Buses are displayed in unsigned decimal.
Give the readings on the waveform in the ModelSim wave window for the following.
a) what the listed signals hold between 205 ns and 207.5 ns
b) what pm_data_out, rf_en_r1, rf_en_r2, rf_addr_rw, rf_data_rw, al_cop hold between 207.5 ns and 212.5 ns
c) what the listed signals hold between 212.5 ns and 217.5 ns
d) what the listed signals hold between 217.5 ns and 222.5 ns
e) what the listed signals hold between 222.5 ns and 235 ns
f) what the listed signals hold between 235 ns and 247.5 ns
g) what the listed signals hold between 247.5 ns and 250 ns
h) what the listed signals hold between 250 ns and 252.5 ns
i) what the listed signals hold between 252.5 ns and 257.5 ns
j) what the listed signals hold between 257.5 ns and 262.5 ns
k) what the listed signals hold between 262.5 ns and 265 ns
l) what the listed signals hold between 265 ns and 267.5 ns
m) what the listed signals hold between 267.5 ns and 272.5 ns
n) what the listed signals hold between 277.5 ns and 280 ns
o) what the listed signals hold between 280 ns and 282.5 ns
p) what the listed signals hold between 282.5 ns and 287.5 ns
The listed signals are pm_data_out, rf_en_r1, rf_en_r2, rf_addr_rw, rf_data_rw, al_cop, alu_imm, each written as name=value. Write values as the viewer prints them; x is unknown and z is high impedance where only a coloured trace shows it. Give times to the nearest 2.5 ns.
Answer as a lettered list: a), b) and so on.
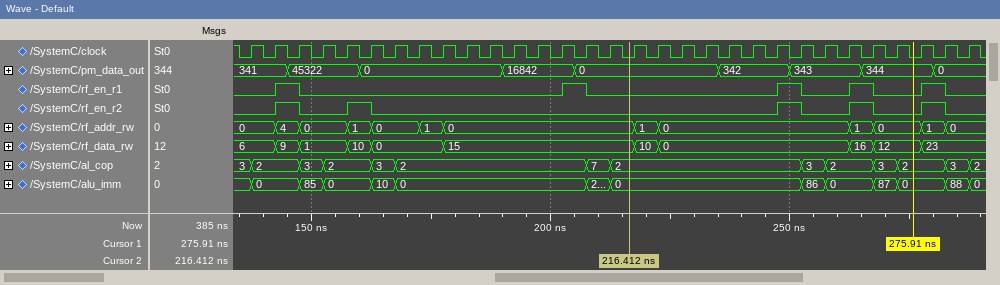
a) pm_data_out=0, rf_en_r1=1, rf_en_r2=0, rf_addr_rw=0, rf_data_rw=15, al_cop=2, alu_imm=0
b) pm_data_out=0, rf_en_r1=0, rf_en_r2=0, rf_addr_rw=0, rf_data_rw=15, al_cop=7
c) pm_data_out=0, rf_en_r1=0, rf_en_r2=0, rf_addr_rw=0, rf_data_rw=15, al_cop=2, alu_imm=0
d) pm_data_out=0, rf_en_r1=0, rf_en_r2=0, rf_addr_rw=1, rf_data_rw=10, al_cop=2, alu_imm=0
e) pm_data_out=0, rf_en_r1=0, rf_en_r2=0, rf_addr_rw=0, rf_data_rw=0, al_cop=2, alu_imm=0
f) pm_data_out=342, rf_en_r1=0, rf_en_r2=0, rf_addr_rw=0, rf_data_rw=0, al_cop=2, alu_imm=0
g) pm_data_out=342, rf_en_r1=1, rf_en_r2=1, rf_addr_rw=0, rf_data_rw=0, al_cop=2, alu_imm=0
h) pm_data_out=343, rf_en_r1=1, rf_en_r2=1, rf_addr_rw=0, rf_data_rw=0, al_cop=2, alu_imm=0
i) pm_data_out=343, rf_en_r1=0, rf_en_r2=0, rf_addr_rw=0, rf_data_rw=0, al_cop=3, alu_imm=86
j) pm_data_out=343, rf_en_r1=0, rf_en_r2=0, rf_addr_rw=0, rf_data_rw=0, al_cop=2, alu_imm=0
k) pm_data_out=343, rf_en_r1=1, rf_en_r2=1, rf_addr_rw=1, rf_data_rw=16, al_cop=2, alu_imm=0
l) pm_data_out=344, rf_en_r1=1, rf_en_r2=1, rf_addr_rw=1, rf_data_rw=16, al_cop=2, alu_imm=0
m) pm_data_out=344, rf_en_r1=0, rf_en_r2=0, rf_addr_rw=0, rf_data_rw=12, al_cop=3, alu_imm=87
n) pm_data_out=344, rf_en_r1=1, rf_en_r2=1, rf_addr_rw=1, rf_data_rw=23, al_cop=2, alu_imm=0
o) pm_data_out=0, rf_en_r1=1, rf_en_r2=1, rf_addr_rw=1, rf_data_rw=23, al_cop=2, alu_imm=0
p) pm_data_out=0, rf_en_r1=0, rf_en_r2=0, rf_addr_rw=0, rf_data_rw=23, al_cop=3, alu_imm=88
